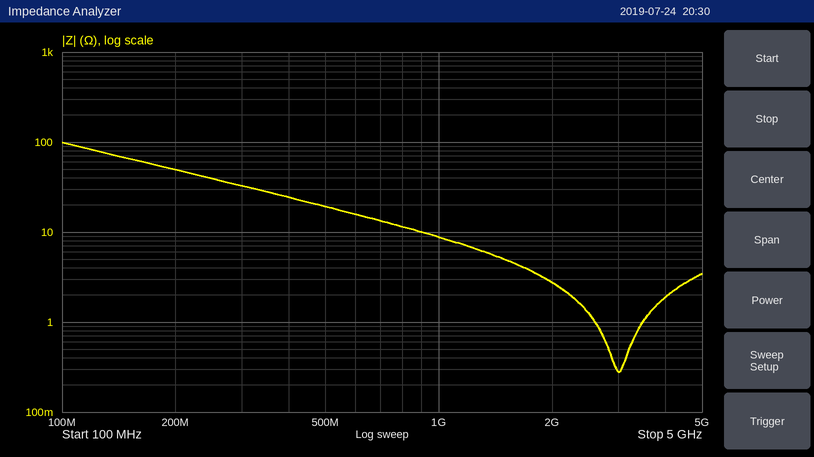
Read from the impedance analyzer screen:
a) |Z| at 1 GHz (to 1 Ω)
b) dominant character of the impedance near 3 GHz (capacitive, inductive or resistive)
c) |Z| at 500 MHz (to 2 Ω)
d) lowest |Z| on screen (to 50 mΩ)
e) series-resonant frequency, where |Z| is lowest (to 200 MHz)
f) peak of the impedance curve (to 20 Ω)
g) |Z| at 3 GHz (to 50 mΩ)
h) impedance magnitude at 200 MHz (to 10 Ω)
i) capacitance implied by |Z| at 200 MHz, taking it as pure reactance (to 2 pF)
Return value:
9 Ω
resistive
20 Ω
300 mΩ
3.0 GHz
100 Ω
300 mΩ
50 Ω
16 pF
